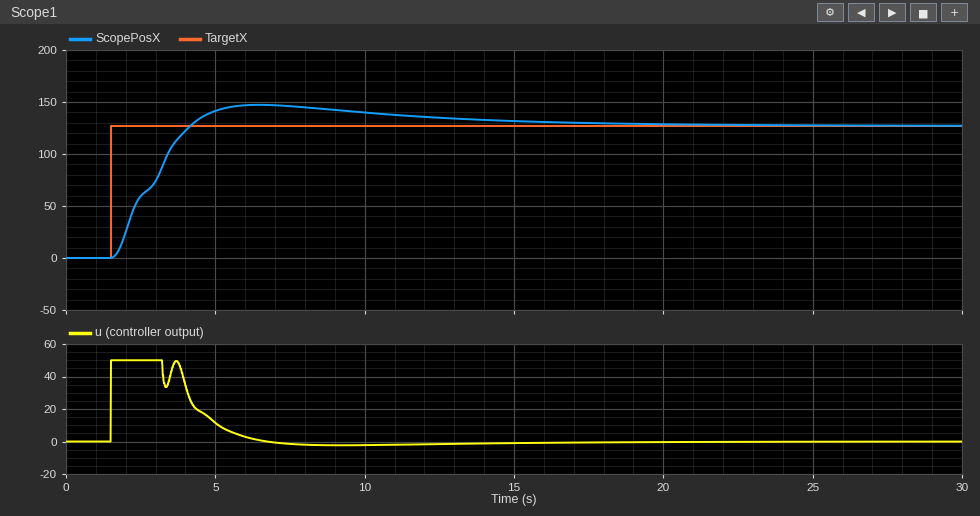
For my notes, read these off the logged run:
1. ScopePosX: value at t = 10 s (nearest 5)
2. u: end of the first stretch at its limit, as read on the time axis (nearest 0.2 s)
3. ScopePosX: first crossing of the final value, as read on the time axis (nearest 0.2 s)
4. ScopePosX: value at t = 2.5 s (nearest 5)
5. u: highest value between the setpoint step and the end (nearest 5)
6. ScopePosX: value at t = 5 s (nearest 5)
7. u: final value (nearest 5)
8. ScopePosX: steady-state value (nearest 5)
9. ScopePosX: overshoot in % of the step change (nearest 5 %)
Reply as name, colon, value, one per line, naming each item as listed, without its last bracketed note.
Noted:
ScopePosX: value at t = 10 s: 140
u: end of the first stretch at its limit, as read on the time axis: 3.2 s
ScopePosX: first crossing of the final value, as read on the time axis: 4.2 s
ScopePosX: value at t = 2.5 s: 60
u: highest value between the setpoint step and the end: 50
ScopePosX: value at t = 5 s: 140
u: final value: 0
ScopePosX: steady-state value: 125
ScopePosX: overshoot in % of the step change: 15 %
